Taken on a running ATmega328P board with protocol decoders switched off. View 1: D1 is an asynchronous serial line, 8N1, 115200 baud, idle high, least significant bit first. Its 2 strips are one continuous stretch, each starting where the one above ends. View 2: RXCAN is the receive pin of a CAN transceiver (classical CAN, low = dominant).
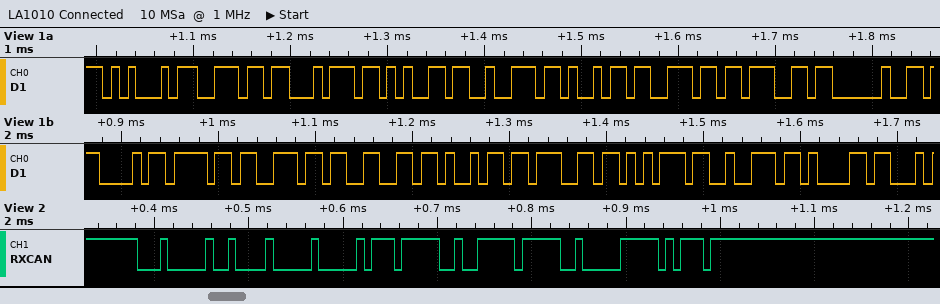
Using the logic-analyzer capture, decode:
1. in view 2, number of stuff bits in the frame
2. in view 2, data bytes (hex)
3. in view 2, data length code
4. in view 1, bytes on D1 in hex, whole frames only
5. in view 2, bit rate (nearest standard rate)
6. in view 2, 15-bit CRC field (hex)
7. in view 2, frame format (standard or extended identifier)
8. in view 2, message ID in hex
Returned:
8
00 77 D3 FF
4
45 6E 74 65 72 69 6E 67 20 43 6F 6E 66 69 67 75 72 61
125 kbit/s
0x20FB
standard
0x101
